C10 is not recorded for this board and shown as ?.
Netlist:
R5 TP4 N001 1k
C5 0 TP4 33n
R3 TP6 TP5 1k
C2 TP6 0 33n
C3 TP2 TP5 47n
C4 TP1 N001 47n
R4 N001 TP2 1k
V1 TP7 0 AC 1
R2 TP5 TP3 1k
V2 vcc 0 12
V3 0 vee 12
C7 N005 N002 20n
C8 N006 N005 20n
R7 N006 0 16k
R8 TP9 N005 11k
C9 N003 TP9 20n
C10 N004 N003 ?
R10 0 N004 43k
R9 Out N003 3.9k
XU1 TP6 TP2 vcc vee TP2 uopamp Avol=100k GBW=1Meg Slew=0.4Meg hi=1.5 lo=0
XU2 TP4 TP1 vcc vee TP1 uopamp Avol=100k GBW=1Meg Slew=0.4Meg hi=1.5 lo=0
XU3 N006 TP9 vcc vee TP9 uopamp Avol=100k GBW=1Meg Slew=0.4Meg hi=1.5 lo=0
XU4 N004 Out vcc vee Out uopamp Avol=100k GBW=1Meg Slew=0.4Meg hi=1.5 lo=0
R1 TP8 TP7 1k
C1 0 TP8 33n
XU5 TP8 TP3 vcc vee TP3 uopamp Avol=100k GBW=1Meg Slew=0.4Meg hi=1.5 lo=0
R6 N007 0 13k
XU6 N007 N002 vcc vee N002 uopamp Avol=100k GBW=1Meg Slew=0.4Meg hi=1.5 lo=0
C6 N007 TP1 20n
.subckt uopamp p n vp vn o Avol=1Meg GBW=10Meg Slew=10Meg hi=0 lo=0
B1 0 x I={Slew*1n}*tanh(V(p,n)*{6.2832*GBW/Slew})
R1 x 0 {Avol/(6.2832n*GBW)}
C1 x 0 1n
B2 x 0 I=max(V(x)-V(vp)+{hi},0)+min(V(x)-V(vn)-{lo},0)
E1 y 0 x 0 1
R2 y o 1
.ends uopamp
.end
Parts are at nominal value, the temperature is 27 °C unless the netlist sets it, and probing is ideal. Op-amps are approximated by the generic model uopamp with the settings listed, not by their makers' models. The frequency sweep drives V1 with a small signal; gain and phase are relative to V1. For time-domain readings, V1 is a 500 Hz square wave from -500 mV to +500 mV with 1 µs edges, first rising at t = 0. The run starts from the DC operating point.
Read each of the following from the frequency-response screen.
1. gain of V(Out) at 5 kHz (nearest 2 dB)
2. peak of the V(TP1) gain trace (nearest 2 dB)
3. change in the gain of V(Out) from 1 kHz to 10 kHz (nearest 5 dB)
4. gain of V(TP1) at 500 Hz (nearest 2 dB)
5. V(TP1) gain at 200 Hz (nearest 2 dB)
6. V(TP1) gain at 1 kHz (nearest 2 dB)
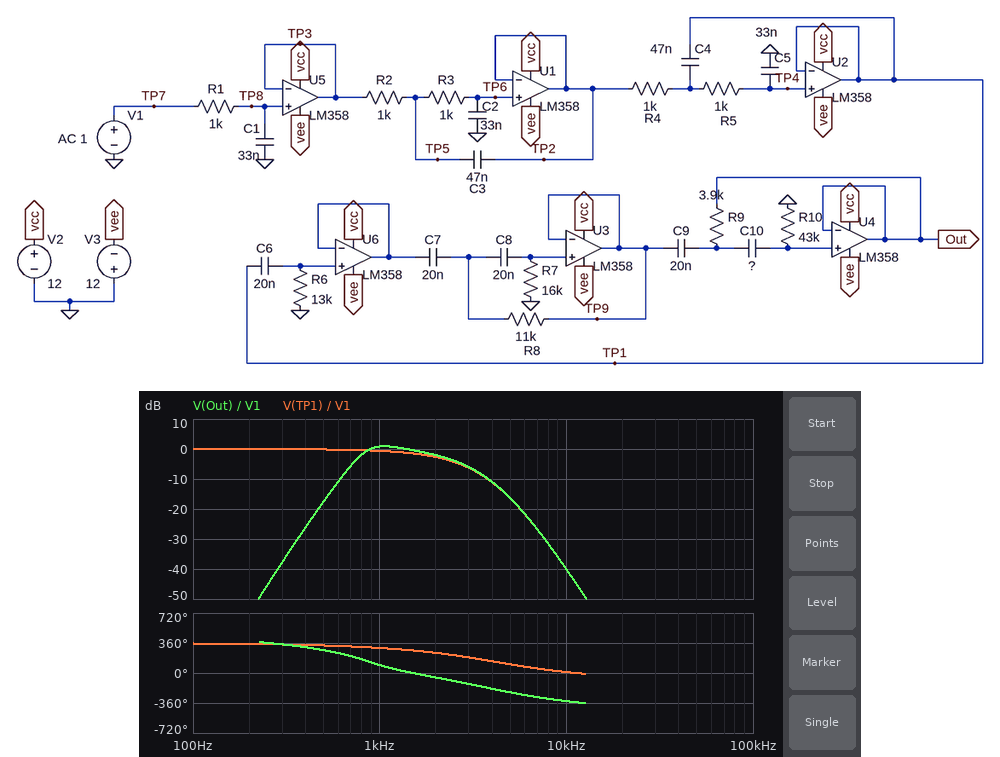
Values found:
-16 dB
0 dB
-40 dB
0 dB
0 dB
0 dB
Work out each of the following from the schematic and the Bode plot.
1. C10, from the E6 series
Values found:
10 nF
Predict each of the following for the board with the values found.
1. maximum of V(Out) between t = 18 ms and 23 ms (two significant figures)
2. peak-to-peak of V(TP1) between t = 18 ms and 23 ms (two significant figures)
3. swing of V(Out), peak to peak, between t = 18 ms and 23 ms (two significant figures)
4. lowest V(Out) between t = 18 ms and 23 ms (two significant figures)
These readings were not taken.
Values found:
260 mV
1.0 V
530 mV
-260 mV
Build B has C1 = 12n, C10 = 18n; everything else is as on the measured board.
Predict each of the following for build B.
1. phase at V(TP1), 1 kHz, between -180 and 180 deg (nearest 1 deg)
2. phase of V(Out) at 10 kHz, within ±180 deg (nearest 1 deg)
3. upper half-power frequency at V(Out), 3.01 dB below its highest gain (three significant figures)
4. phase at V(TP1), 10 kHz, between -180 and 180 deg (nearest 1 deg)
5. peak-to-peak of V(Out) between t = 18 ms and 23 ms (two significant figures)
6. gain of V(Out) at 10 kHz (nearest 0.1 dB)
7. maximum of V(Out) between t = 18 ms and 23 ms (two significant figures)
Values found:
-52 deg
49 deg
2.42 kHz
39 deg
590 mV
-34.8 dB
290 mV
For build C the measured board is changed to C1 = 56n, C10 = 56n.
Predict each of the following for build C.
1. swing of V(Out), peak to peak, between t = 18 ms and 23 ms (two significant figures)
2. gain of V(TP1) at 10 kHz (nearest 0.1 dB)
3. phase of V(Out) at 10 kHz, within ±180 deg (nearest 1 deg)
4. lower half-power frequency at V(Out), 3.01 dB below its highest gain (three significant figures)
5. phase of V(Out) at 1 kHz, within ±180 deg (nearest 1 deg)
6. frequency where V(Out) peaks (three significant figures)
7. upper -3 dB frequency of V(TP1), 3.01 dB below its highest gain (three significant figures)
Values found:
830 mV
-44.1 dB
11 deg
574 Hz
37 deg
1.20 kHz
1.79 kHz
